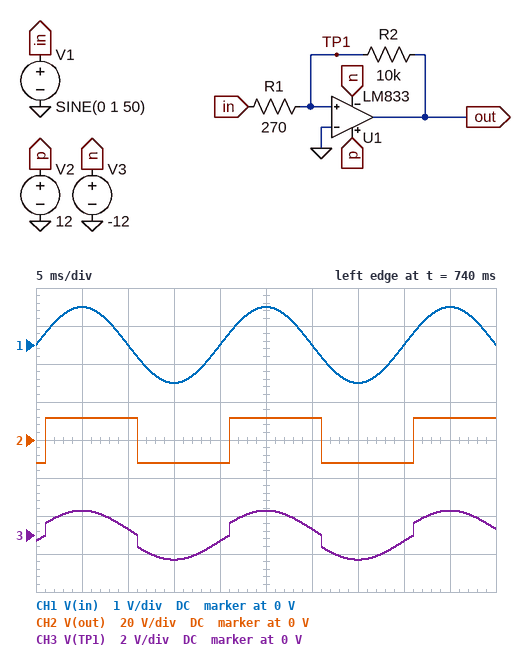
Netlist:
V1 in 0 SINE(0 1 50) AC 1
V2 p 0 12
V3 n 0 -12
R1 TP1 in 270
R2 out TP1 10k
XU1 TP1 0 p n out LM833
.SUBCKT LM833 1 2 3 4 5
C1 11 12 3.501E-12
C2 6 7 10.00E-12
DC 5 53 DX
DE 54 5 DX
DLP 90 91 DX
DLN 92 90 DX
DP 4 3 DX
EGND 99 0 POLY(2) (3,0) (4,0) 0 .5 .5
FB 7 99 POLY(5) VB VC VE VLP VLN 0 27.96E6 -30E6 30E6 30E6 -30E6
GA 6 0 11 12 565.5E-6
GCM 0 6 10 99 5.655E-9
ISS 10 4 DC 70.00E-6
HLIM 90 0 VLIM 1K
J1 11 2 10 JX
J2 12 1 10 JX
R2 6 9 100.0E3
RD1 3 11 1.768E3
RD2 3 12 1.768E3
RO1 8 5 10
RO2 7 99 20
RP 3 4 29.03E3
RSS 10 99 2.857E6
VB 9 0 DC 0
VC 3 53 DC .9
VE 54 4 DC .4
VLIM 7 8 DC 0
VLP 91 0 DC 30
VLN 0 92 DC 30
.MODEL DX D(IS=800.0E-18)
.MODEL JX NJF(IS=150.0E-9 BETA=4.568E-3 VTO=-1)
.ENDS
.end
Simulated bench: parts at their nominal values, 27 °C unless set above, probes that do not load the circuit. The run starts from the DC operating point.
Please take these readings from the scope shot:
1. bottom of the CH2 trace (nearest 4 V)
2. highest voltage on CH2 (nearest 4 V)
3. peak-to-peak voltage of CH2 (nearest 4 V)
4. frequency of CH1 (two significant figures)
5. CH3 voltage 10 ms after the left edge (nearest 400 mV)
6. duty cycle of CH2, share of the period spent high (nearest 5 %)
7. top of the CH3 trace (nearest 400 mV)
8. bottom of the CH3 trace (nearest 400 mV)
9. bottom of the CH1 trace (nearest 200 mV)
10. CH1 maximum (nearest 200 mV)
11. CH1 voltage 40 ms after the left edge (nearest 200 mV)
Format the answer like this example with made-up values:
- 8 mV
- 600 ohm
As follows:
- -12 V
- 12 V
- 24 V
- 50 Hz
- 400 mV
- 50 %
- 1.2 V
- -1.2 V
- -1.0 V
- 1.0 V
- 0 V
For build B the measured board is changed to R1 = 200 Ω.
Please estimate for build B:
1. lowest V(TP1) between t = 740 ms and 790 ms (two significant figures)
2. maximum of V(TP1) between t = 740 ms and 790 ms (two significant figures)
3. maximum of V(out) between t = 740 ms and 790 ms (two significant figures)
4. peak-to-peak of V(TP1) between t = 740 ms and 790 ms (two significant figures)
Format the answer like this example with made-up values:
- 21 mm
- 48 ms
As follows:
- -1.2 V
- 1.2 V
- 12 V
- 2.4 V
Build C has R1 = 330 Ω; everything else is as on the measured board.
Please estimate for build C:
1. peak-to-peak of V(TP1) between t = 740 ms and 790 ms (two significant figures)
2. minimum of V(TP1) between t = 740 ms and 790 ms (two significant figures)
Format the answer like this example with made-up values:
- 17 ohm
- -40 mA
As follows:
- 2.7 V
- -1.4 V
